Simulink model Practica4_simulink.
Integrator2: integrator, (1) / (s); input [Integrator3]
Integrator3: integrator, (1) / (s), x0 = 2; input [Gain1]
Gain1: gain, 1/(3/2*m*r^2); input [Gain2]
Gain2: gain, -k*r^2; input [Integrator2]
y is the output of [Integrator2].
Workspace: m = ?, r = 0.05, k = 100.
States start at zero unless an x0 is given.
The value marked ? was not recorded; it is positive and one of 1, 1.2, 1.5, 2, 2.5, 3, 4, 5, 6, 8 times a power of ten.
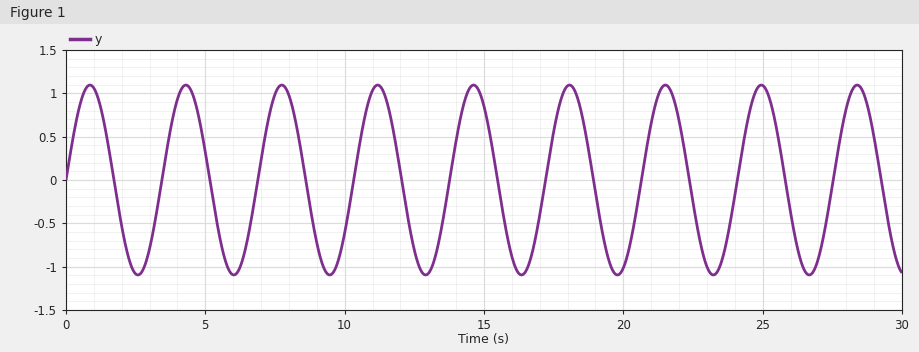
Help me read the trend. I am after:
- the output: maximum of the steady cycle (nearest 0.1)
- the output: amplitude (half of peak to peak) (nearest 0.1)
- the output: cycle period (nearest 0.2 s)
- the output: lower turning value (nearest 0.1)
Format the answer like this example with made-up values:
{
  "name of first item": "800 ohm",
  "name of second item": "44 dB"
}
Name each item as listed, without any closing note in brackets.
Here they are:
{
  "the output: maximum of the steady cycle": "1.1",
  "the output: amplitude (half of peak to peak)": "1.1",
  "the output: cycle period": "3.4 s",
  "the output: lower turning value": "-1.1"
}
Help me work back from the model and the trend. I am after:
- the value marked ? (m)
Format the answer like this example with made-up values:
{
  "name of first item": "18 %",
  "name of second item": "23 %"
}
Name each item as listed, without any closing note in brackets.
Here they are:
{
  "the value marked ?": "20"
}
